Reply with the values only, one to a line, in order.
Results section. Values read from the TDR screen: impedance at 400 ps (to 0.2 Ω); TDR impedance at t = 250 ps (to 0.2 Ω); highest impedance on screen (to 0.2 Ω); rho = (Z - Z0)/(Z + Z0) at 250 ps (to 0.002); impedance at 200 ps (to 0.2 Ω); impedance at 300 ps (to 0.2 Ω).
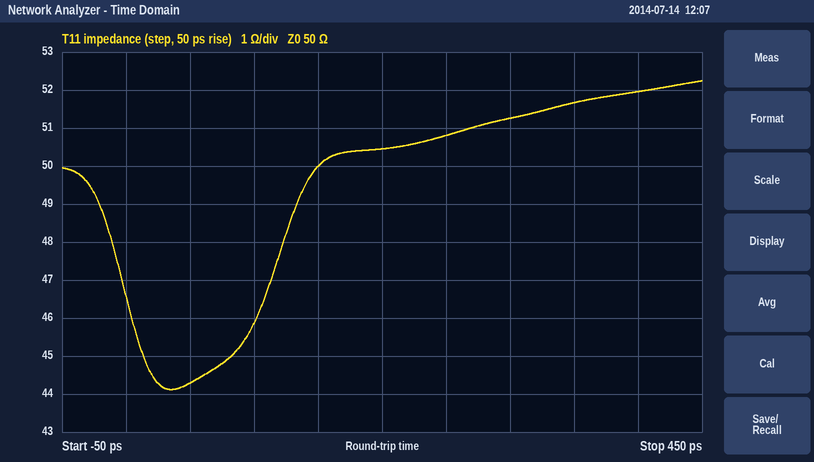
52.0 Ω
50.8 Ω
52.2 Ω
+0.008
50.4 Ω
51.2 Ω
